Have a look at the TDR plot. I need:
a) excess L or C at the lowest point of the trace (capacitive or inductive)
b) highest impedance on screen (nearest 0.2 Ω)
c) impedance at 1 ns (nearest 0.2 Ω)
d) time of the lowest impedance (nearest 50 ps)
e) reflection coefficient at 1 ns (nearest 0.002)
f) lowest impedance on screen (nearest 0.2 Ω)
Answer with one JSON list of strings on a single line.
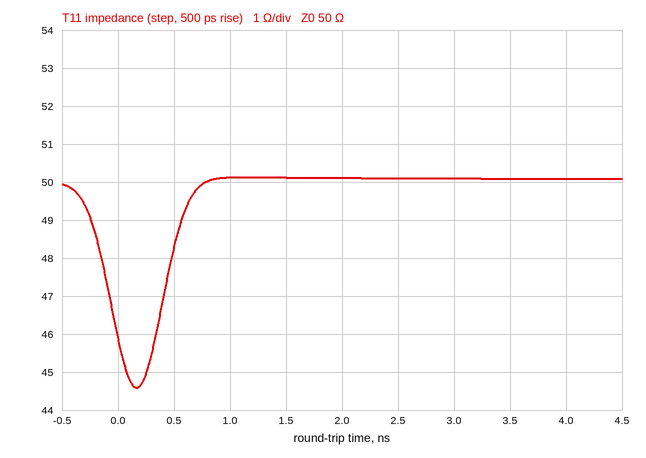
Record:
["capacitive", "50.2 Ω", "50.2 Ω", "150 ps", "+0.002", "44.6 Ω"]
